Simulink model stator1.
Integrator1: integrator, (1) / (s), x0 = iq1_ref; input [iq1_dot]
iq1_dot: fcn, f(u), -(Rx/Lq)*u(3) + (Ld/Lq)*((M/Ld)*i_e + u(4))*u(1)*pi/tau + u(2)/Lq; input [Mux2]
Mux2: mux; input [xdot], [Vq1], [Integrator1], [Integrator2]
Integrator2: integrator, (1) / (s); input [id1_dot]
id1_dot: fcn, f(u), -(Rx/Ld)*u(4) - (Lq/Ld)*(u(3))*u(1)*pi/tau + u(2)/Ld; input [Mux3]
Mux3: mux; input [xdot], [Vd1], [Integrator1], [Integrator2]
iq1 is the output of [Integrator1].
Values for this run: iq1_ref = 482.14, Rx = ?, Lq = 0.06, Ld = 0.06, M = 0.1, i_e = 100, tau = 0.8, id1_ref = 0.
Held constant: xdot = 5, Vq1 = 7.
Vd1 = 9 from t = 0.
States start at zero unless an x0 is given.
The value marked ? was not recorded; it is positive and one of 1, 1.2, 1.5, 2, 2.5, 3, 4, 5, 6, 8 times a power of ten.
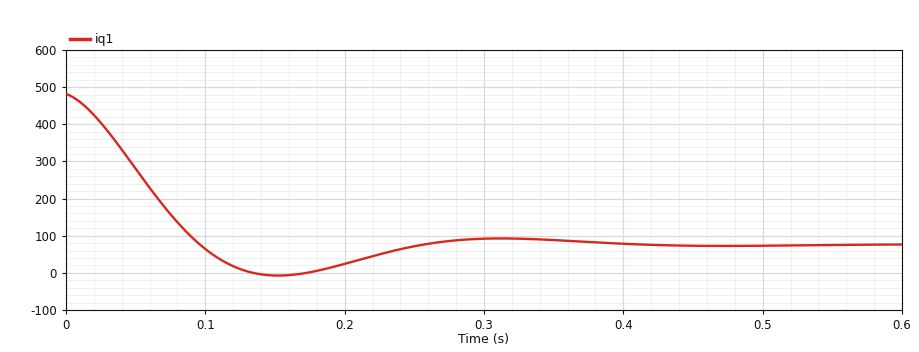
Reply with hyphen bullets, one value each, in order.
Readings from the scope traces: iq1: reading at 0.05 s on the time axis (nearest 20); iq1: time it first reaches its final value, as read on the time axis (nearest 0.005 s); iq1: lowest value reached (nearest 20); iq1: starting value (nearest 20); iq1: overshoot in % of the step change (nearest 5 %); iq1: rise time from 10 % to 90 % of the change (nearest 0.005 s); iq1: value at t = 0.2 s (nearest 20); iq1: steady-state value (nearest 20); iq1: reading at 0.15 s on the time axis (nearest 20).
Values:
- 280
- 0.095 s
- 0
- 480
- 20 %
- 0.070 s
- 20
- 80
- 0
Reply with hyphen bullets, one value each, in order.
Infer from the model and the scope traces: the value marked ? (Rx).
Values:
- 0.6
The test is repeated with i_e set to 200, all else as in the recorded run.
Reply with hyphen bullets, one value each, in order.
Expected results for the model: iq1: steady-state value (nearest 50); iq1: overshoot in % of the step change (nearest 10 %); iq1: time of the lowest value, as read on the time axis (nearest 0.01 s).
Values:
- 150
- 20 %
- 0.17 s
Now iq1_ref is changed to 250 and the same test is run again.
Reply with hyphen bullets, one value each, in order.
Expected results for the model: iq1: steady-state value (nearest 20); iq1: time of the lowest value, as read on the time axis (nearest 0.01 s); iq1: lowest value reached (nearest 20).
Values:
- 80
- 0.17 s
- 40
